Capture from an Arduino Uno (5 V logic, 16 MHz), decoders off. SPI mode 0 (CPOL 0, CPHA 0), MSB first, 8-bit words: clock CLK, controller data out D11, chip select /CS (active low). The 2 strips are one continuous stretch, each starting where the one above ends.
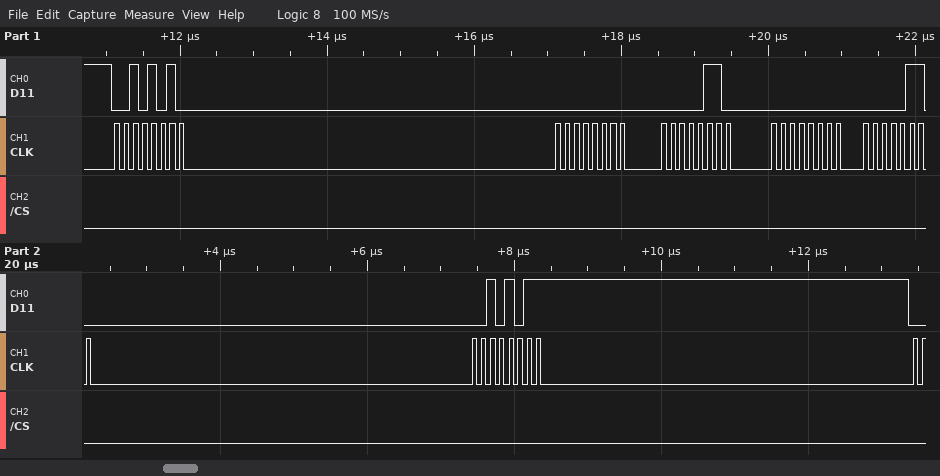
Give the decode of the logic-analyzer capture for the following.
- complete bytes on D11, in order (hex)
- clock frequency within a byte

0x2A 0x00 0x06 0x00 0x06 0x2B
8 MHz
